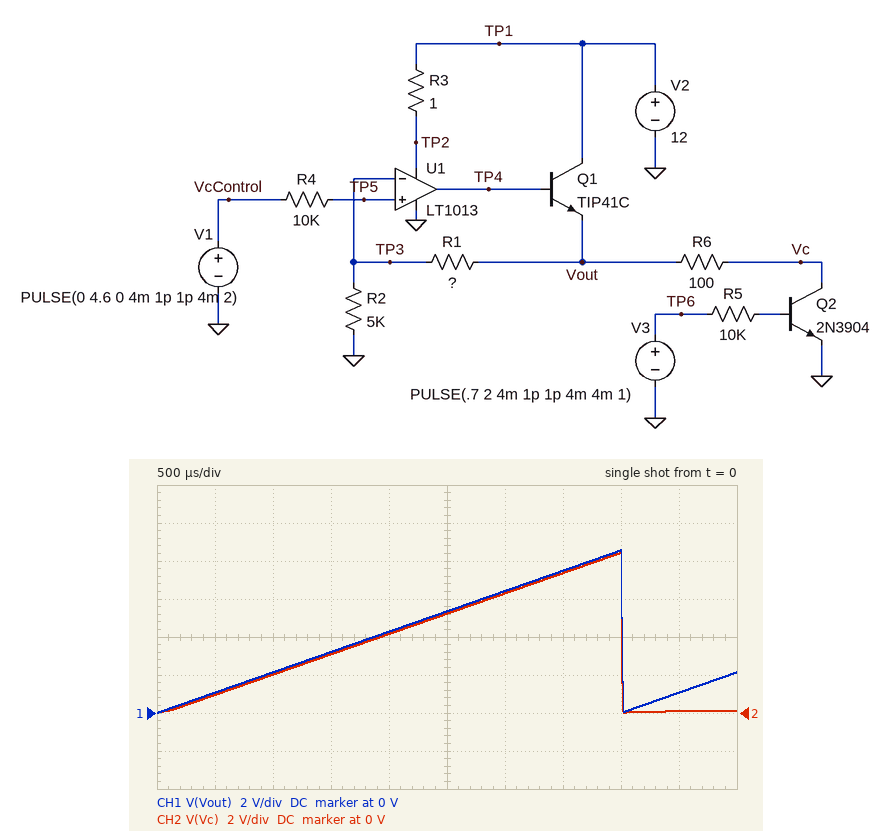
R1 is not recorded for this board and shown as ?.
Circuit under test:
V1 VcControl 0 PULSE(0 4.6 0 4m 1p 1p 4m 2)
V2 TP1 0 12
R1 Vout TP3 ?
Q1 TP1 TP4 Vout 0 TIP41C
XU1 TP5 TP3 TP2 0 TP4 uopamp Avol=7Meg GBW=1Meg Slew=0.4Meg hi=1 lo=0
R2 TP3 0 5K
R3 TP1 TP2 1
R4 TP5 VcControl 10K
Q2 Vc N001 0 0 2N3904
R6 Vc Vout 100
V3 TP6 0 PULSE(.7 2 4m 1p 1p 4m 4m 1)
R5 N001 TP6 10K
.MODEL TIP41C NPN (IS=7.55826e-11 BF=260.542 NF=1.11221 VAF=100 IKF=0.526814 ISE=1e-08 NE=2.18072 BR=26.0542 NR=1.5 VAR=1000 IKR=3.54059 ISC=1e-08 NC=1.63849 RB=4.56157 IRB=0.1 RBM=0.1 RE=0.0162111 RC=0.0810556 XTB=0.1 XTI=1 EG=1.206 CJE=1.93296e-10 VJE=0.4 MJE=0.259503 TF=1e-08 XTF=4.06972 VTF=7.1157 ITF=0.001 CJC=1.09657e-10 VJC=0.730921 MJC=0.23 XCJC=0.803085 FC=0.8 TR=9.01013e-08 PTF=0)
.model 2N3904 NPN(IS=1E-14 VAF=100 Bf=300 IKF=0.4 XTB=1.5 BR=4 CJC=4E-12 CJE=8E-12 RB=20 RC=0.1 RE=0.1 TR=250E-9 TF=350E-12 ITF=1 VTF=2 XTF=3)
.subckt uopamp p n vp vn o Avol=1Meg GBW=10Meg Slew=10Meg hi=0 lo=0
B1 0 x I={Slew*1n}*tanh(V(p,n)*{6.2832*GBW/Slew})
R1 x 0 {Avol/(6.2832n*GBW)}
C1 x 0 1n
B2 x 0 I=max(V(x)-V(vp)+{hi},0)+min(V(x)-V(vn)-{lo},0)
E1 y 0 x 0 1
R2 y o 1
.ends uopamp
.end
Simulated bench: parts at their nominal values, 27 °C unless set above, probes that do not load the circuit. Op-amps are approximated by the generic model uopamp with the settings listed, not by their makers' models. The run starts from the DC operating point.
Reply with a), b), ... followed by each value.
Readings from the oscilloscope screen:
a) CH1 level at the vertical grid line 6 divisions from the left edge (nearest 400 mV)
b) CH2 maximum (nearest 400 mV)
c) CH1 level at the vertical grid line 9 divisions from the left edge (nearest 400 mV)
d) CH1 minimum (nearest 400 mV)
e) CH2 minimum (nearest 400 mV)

a) 6.4 V
b) 8.4 V
c) 1.2 V
d) 0 V
e) 0 V
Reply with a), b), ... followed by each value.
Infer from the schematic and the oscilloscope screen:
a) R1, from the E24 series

a) 4.3 kΩ
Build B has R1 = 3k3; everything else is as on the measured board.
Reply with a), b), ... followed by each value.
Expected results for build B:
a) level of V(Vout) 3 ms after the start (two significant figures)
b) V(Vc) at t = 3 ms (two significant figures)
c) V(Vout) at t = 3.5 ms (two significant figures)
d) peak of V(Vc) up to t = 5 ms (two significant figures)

a) 5.7 V
b) 5.6 V
c) 6.7 V
d) 7.5 V
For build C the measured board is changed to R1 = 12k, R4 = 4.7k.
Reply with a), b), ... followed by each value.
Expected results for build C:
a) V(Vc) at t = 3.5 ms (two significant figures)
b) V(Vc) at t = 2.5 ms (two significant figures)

a) 10 V
b) 9.6 V
